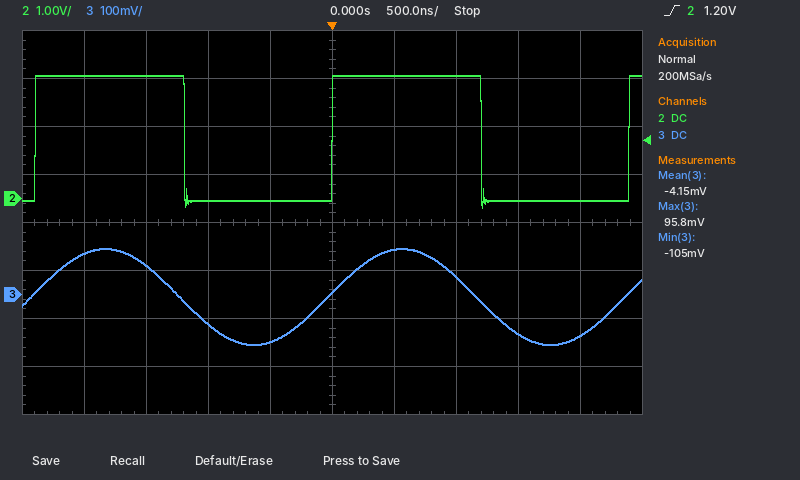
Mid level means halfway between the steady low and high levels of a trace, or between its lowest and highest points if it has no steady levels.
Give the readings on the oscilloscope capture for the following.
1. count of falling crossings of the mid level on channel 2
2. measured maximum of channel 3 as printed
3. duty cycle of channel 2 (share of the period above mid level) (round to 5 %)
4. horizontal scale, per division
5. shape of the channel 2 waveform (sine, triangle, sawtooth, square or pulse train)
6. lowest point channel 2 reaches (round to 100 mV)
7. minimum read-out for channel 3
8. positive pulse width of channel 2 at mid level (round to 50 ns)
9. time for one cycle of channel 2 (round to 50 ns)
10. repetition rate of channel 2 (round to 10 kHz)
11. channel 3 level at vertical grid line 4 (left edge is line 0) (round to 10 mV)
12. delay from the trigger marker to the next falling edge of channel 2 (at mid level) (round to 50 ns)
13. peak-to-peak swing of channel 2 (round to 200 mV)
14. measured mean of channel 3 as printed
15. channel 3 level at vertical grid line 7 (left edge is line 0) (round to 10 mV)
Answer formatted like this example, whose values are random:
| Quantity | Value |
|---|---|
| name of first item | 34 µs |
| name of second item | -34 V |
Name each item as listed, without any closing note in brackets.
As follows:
| Quantity | Value |
|---|---|
| count of falling crossings of the mid level on channel 2 | 2 |
| measured maximum of channel 3 as printed | 95.8 mV |
| duty cycle of channel 2 (share of the period above mid level) | 50 % |
| horizontal scale, per division | 500 ns |
| shape of the channel 2 waveform | square |
| lowest point channel 2 reaches | -200 mV |
| minimum read-out for channel 3 | -105 mV |
| positive pulse width of channel 2 at mid level | 1.20 µs |
| time for one cycle of channel 2 | 2.40 µs |
| repetition rate of channel 2 | 420 kHz |
| channel 3 level at vertical grid line 4 (left edge is line 0) | -100 mV |
| delay from the trigger marker to the next falling edge of channel 2 (at mid level) | 1.20 µs |
| peak-to-peak swing of channel 2 | 2.8 V |
| measured mean of channel 3 as printed | -4.15 mV |
| channel 3 level at vertical grid line 7 (left edge is line 0) | 40 mV |
